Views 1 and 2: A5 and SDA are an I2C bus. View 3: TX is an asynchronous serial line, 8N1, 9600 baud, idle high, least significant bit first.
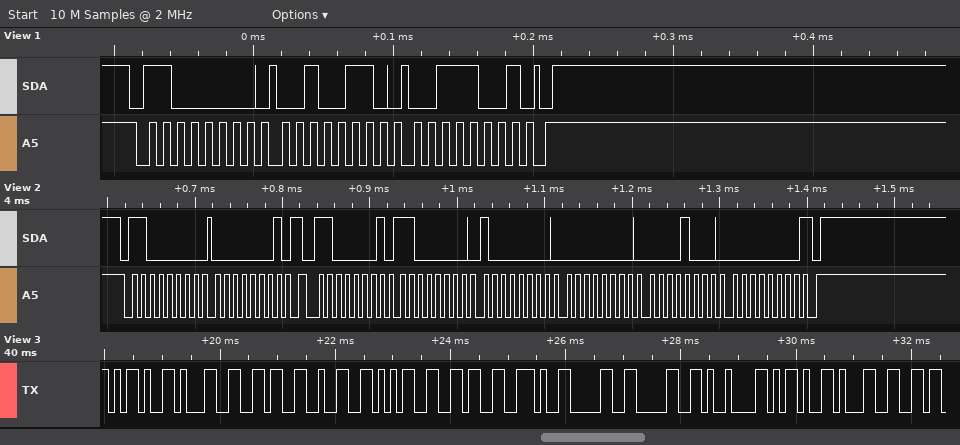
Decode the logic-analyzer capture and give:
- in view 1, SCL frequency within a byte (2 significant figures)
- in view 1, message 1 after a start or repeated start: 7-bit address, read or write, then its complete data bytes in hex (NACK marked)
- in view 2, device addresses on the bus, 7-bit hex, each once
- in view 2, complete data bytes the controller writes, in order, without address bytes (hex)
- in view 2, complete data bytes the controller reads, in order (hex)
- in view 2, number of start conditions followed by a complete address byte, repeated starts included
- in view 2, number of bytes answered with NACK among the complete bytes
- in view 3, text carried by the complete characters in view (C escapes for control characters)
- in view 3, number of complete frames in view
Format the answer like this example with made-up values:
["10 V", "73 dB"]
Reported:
["100 kHz", "0x60 write: 26 39", "0x60", "01", "C0 80 00 08 00", "2", "1", "\"-16256.00\\t-1\"", "12"]
